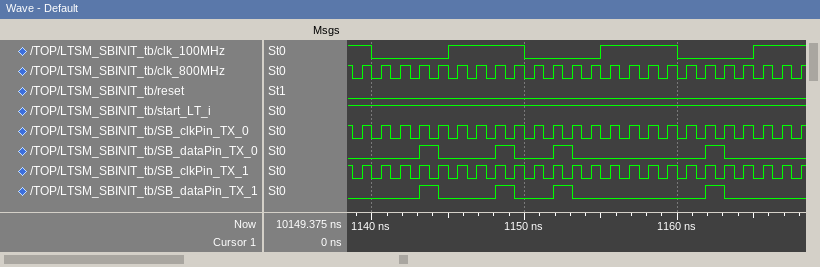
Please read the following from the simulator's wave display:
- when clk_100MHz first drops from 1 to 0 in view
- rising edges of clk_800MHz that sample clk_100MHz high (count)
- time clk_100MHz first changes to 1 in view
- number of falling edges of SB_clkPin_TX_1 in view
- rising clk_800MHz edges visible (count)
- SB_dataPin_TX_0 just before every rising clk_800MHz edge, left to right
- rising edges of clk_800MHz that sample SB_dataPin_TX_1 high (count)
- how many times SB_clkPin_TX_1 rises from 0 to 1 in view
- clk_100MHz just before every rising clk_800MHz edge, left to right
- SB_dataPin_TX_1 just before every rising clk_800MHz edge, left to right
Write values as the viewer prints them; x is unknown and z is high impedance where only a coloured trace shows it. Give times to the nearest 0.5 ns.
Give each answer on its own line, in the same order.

1140 ns
12
1145 ns
24
24
0 0 0 0 1 0 0 0 1 0 0 1 0 0 0 0 0 0 0 1 0 0 0 0
4
24
1 0 0 0 0 1 1 1 1 0 0 0 0 1 1 1 1 0 0 0 0 1 1 1
0 0 0 0 1 0 0 0 1 0 0 1 0 0 0 0 0 0 0 1 0 0 0 0
